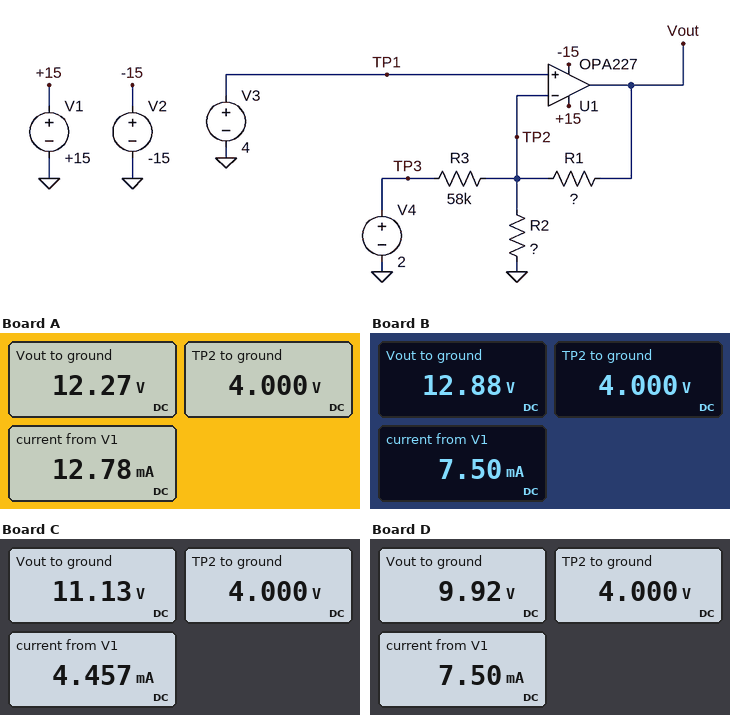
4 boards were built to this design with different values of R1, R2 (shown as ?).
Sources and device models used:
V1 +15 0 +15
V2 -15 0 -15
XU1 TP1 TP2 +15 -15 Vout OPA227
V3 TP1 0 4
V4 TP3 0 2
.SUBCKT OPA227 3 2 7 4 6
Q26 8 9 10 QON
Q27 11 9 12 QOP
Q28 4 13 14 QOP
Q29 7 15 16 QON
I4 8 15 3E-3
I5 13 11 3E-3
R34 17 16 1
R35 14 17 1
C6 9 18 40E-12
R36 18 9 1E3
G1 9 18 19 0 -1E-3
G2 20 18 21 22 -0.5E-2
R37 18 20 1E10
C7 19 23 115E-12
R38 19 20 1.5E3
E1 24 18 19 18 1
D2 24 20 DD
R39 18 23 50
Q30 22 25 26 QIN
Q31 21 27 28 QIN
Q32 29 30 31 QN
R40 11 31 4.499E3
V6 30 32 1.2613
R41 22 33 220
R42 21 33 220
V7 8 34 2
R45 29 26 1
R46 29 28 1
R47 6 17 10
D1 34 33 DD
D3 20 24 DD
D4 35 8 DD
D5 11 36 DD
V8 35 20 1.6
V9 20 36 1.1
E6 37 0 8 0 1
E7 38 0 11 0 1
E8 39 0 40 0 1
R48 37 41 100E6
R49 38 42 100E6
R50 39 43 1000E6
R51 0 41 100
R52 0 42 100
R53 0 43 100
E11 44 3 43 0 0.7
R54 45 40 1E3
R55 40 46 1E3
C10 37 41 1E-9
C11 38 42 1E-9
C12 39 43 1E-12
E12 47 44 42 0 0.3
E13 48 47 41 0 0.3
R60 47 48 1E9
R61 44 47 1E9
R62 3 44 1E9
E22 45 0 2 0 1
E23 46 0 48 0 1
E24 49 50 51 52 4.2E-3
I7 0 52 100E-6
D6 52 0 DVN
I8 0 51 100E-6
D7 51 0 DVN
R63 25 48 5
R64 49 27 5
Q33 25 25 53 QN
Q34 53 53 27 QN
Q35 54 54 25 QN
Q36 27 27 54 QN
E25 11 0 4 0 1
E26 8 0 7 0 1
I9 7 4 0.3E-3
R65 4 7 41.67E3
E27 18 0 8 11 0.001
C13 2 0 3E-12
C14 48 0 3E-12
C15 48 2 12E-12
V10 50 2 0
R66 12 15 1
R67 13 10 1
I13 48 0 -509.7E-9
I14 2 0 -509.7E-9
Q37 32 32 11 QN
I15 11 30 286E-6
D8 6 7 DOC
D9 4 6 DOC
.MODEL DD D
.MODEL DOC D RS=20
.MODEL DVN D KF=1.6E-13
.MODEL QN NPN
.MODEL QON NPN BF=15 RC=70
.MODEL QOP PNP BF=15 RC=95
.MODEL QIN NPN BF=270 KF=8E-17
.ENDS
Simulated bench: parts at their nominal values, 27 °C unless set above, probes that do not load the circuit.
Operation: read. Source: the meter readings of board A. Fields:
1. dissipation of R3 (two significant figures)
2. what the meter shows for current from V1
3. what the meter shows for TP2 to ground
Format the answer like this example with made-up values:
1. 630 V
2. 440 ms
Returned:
1. 69 µW
2. 12.78 mA
3. 4.000 V
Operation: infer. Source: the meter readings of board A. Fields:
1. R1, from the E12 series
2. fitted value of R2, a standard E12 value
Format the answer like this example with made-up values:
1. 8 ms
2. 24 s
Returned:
1. 680 Ω
2. 330 Ω
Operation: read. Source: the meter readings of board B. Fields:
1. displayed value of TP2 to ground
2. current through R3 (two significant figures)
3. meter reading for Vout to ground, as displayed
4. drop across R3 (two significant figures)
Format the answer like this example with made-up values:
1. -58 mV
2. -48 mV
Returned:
1. 4.000 V
2. 34 µA
3. 12.88 V
4. 2.0 V
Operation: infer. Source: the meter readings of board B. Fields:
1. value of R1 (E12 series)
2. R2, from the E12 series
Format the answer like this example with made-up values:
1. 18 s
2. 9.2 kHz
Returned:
1. 1.5 kΩ
2. 680 Ω
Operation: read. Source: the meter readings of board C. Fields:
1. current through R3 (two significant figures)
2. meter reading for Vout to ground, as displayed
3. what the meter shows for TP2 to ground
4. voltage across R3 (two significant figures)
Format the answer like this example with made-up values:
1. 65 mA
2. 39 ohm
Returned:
1. 34 µA
2. 11.13 V
3. 4.000 V
4. 2.0 V
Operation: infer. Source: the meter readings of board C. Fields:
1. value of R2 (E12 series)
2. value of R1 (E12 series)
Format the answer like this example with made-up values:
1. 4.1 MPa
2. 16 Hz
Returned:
1. 2.7 kΩ
2. 4.7 kΩ
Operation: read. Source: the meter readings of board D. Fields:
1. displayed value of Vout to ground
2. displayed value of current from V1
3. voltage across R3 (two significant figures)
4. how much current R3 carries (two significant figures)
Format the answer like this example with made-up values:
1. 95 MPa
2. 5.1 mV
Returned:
1. 9.92 V
2. 7.50 mA
3. 2.0 V
4. 34 µA
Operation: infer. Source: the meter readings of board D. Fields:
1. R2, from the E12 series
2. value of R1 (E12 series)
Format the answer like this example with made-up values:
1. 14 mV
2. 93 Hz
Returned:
1. 680 Ω
2. 1 kΩ
